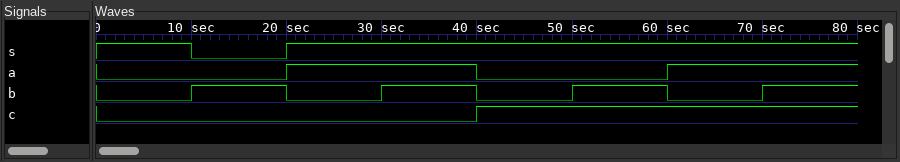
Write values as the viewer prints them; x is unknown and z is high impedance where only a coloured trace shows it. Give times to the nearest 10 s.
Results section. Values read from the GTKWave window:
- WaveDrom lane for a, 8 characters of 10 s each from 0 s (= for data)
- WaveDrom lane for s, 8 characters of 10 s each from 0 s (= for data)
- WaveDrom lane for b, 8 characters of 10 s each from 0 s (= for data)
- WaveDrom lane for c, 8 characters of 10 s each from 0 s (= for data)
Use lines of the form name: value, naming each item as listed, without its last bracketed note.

WaveDrom lane for a, 8 characters of 10 s each from 0 s: {name: 'a', wave: '0.1.0.1.'}
WaveDrom lane for s, 8 characters of 10 s each from 0 s: {name: 's', wave: '101.....'}
WaveDrom lane for b, 8 characters of 10 s each from 0 s: {name: 'b', wave: '01010101'}
WaveDrom lane for c, 8 characters of 10 s each from 0 s: {name: 'c', wave: '0...1...'}
